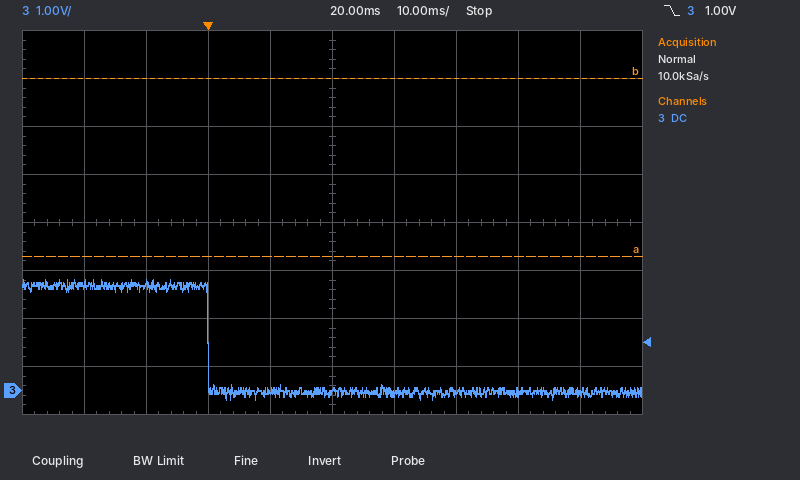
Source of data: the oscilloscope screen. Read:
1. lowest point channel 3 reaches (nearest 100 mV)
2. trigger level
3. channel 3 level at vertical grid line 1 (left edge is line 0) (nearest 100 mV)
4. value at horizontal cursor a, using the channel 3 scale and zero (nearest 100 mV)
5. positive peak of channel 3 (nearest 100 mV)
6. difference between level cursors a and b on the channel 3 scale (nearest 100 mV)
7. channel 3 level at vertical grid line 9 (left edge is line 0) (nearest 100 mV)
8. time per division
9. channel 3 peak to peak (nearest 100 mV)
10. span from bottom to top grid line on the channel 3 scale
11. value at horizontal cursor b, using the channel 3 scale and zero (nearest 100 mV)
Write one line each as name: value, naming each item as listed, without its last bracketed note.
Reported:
lowest point channel 3 reaches: -200 mV
trigger level: 1.00 V
channel 3 level at vertical grid line 1 (left edge is line 0): 2.2 V
value at horizontal cursor a, using the channel 3 scale and zero: 2.8 V
positive peak of channel 3: 2.3 V
difference between level cursors a and b on the channel 3 scale: 3.7 V
channel 3 level at vertical grid line 9 (left edge is line 0): 0.0 V
time per division: 10 ms
channel 3 peak to peak: 2.5 V
span from bottom to top grid line on the channel 3 scale: 8 V
value at horizontal cursor b, using the channel 3 scale and zero: 6.5 V
